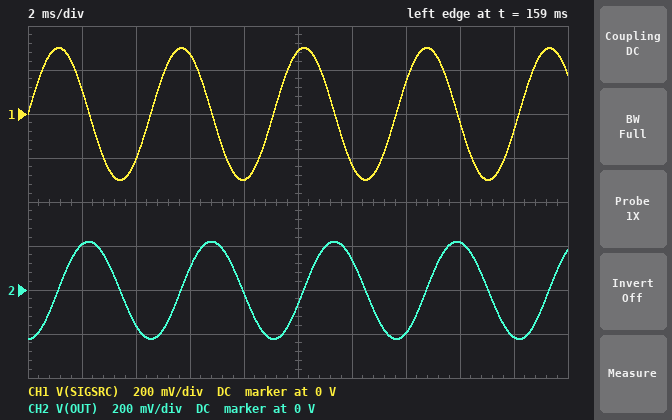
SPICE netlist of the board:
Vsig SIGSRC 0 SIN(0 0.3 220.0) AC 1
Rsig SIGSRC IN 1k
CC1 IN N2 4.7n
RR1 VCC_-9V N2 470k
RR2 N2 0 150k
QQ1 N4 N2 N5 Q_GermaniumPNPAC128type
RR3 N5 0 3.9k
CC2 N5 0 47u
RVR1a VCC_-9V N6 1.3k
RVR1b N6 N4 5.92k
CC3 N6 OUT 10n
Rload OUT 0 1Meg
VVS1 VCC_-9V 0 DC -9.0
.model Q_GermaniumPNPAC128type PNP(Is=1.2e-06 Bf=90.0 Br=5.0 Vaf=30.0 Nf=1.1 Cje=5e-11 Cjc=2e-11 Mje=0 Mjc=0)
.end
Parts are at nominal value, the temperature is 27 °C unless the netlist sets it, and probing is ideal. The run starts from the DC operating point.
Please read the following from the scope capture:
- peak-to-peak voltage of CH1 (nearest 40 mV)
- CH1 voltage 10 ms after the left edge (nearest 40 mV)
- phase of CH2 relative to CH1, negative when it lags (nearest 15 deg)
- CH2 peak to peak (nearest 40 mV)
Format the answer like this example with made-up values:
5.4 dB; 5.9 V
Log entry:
600 mV; 280 mV; -90 deg; 440 mV
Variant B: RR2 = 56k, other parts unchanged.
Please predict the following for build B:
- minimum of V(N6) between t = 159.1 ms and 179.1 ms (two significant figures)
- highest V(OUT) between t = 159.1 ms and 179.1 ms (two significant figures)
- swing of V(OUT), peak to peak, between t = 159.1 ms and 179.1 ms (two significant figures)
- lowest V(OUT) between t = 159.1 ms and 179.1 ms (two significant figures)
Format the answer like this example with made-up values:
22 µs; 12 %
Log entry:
-8.9 V; 200 mV; 380 mV; -180 mV
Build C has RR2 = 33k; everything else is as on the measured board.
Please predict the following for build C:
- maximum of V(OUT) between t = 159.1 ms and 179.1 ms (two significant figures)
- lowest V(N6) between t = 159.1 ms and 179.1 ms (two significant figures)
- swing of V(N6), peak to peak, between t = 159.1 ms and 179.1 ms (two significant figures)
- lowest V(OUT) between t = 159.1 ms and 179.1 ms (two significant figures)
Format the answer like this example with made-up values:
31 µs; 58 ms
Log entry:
150 mV; -9.0 V; 260 mV; -110 mV
